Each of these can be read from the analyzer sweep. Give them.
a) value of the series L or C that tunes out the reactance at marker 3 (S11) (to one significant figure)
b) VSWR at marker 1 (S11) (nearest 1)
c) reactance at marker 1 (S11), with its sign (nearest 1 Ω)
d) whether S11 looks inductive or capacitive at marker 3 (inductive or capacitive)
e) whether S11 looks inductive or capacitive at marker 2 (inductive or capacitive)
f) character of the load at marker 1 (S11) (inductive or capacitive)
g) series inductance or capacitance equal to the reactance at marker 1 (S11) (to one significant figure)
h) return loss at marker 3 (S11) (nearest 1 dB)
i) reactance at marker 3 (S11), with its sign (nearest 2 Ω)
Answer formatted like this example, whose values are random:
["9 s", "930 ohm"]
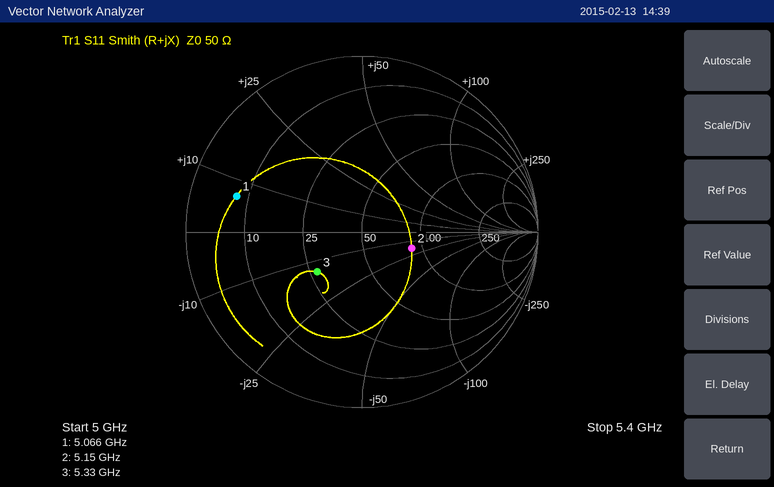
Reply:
["400 pH", "7", "+7 Ω", "capacitive", "capacitive", "inductive", "200 pH", "9 dB", "-14 Ω"]
